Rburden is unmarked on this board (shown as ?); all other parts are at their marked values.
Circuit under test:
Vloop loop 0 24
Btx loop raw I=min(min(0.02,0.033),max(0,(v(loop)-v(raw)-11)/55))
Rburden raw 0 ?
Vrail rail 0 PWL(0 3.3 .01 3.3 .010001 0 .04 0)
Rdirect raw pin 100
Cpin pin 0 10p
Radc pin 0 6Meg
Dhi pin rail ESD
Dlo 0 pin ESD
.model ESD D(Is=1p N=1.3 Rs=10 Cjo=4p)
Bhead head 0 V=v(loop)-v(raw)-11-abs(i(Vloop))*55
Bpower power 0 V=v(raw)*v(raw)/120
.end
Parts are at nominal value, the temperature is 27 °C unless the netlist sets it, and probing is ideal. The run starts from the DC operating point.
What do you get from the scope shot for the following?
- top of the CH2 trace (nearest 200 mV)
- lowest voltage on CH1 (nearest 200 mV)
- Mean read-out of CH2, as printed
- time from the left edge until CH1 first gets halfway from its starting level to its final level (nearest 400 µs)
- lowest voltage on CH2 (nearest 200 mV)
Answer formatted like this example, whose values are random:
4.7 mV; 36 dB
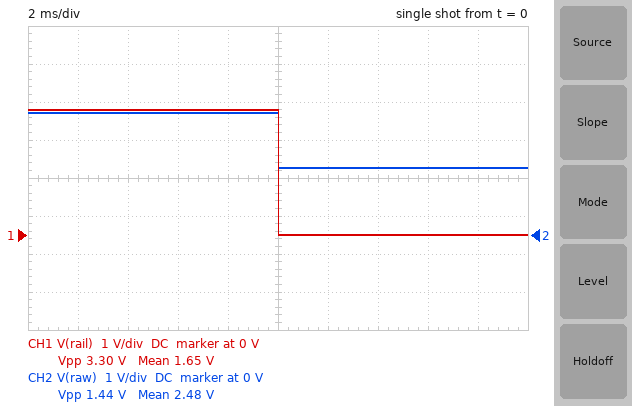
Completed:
3.2 V; 0 V; 2.48 V; 10.0 ms; 1.8 V
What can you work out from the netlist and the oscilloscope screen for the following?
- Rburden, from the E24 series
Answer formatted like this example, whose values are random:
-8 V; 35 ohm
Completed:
160 Ω
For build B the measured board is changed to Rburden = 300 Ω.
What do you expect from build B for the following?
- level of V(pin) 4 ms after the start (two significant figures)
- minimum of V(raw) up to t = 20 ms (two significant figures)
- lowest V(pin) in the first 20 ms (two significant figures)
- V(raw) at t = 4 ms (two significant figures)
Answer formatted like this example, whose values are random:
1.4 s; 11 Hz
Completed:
4.1 V; 2.2 V; 910 mV; 4.6 V
